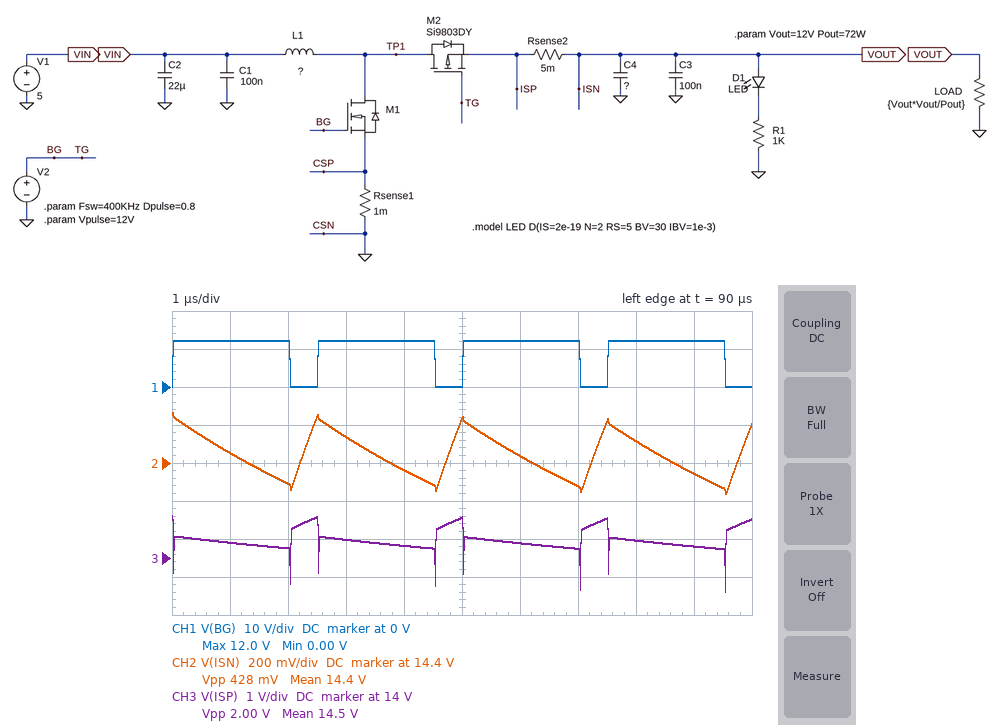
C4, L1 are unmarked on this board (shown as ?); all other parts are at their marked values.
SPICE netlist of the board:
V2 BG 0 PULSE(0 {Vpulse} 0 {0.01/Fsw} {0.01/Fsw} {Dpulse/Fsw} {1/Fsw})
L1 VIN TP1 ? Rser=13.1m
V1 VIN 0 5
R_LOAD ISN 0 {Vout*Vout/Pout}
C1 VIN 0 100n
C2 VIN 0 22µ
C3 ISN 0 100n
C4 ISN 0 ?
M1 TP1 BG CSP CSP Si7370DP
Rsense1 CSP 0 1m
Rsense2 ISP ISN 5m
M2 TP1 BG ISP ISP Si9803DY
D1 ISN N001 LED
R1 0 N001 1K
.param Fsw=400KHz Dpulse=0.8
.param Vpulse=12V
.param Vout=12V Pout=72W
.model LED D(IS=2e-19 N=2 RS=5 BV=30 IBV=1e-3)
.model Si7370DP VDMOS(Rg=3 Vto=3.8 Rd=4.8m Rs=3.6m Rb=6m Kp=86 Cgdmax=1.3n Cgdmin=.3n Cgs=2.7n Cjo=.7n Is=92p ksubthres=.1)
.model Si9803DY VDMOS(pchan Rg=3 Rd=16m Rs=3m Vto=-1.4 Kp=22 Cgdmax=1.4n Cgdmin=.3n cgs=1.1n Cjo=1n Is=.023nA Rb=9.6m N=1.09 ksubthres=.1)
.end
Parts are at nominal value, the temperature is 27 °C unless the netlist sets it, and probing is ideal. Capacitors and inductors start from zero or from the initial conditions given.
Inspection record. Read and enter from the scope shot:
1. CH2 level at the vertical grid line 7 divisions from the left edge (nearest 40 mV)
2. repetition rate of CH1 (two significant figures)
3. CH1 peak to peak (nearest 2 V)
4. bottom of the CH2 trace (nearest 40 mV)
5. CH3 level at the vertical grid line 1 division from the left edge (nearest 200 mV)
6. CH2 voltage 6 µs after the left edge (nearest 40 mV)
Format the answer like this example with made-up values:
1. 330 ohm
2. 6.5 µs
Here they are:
1. 14.28 V
2. 400 kHz
3. 12 V
4. 14.24 V
5. 14.4 V
6. 14.44 V
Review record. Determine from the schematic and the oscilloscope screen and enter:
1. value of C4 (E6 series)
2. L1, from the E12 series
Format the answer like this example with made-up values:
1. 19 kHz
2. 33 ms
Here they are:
1. 100 µF
2. 390 nH
